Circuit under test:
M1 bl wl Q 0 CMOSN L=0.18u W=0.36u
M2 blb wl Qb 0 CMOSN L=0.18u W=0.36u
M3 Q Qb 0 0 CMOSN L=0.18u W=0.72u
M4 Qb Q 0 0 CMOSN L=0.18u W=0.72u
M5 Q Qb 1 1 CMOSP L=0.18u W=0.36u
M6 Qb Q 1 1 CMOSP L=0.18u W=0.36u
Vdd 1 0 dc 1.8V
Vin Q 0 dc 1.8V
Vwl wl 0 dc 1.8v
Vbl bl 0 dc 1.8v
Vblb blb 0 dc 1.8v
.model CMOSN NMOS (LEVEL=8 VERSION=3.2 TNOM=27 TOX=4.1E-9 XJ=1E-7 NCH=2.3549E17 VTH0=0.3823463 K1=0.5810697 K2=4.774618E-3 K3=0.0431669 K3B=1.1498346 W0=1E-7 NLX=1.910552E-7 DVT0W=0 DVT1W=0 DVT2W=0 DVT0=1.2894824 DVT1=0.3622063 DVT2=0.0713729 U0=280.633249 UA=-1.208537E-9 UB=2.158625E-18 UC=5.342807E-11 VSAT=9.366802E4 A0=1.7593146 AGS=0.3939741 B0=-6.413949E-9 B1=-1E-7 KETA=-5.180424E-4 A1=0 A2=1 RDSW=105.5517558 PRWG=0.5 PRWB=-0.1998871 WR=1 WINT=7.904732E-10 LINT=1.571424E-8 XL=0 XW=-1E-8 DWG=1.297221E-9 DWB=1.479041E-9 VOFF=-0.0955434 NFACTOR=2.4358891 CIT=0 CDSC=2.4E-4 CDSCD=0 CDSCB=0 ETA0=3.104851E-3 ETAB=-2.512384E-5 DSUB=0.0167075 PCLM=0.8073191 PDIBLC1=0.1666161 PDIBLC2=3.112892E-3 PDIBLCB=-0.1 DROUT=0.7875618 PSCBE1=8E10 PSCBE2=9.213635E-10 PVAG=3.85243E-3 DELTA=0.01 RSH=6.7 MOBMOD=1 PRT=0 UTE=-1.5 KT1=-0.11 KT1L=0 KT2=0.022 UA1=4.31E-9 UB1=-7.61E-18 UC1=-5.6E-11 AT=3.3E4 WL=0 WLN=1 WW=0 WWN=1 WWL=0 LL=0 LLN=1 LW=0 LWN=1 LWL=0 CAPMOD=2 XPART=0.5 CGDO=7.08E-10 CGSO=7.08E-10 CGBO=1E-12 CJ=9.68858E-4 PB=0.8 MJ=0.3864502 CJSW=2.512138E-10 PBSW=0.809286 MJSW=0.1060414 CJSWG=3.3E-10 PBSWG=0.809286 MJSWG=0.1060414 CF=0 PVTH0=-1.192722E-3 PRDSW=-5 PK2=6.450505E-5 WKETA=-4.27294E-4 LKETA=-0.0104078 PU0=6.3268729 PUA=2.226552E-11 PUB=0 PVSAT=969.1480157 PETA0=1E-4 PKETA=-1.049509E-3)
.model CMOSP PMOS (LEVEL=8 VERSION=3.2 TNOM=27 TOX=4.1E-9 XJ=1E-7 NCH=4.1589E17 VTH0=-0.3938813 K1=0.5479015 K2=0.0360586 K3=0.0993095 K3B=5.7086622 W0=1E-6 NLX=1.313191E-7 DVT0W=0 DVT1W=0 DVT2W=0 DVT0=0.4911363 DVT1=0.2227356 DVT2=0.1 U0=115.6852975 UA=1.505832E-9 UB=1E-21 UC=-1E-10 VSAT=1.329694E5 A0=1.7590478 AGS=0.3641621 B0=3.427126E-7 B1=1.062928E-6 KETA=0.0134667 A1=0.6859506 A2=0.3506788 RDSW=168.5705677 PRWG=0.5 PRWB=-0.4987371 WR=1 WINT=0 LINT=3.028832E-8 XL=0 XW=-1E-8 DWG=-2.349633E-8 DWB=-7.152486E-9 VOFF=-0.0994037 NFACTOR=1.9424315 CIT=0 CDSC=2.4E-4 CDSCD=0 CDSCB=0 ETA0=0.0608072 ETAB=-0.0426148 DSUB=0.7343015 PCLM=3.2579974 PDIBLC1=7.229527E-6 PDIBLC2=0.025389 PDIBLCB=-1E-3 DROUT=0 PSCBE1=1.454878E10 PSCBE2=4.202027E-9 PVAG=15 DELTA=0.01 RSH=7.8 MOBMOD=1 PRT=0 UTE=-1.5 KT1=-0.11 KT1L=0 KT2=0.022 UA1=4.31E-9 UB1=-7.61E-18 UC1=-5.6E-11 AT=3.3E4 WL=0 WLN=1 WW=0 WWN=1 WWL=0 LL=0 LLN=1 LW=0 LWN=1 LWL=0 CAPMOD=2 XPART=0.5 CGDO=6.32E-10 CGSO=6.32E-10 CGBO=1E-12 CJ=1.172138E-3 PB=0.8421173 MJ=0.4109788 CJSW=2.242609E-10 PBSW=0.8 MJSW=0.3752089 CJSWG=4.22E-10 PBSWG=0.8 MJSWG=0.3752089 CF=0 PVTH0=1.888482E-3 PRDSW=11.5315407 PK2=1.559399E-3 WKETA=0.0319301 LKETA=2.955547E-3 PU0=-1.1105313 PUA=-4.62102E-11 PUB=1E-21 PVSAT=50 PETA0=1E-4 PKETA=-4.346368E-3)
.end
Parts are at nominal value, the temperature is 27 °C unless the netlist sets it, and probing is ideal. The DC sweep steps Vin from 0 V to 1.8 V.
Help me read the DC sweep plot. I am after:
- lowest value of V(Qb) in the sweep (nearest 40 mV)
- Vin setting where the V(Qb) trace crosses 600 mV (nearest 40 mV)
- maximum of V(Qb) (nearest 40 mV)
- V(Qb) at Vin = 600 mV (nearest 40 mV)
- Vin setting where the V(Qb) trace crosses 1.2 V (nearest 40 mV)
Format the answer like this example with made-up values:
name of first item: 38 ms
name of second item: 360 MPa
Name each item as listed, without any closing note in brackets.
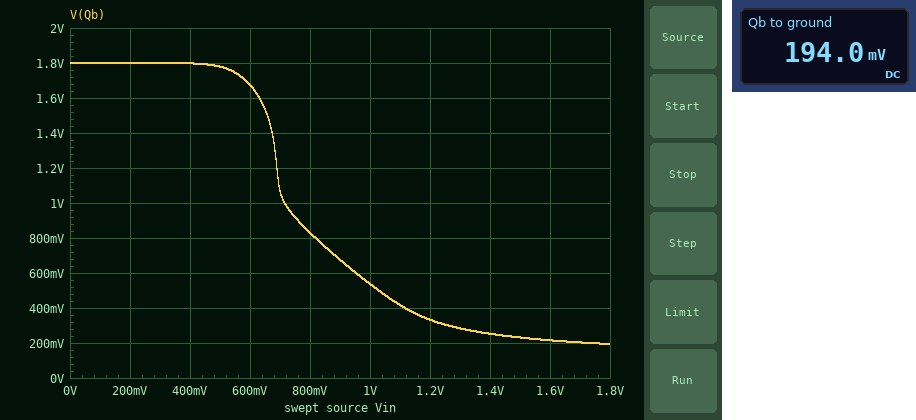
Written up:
lowest value of V(Qb) in the sweep: 200 mV
Vin setting where the V(Qb) trace crosses 600 mV: 960 mV
maximum of V(Qb): 1.80 V
V(Qb) at Vin = 600 mV: 1.68 V
Vin setting where the V(Qb) trace crosses 1.2 V: 680 mV
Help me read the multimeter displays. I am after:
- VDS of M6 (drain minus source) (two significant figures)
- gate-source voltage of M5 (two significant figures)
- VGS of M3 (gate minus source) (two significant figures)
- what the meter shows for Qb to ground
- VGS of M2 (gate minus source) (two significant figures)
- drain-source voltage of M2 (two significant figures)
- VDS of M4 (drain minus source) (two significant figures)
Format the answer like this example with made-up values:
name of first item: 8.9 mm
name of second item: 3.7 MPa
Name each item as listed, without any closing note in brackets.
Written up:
VDS of M6 (drain minus source): -1.6 V
gate-source voltage of M5: -1.6 V
VGS of M3 (gate minus source): 190 mV
what the meter shows for Qb to ground: 194.0 mV
VGS of M2 (gate minus source): 1.6 V
drain-source voltage of M2: 1.6 V
VDS of M4 (drain minus source): 190 mV
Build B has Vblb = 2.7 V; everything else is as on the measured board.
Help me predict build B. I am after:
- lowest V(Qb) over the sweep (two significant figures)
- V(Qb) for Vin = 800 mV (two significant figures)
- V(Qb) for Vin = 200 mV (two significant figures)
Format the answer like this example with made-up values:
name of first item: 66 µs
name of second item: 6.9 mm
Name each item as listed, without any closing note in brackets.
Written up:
lowest V(Qb) over the sweep: 200 mV
V(Qb) for Vin = 800 mV: 860 mV
V(Qb) for Vin = 200 mV: 1.8 V
